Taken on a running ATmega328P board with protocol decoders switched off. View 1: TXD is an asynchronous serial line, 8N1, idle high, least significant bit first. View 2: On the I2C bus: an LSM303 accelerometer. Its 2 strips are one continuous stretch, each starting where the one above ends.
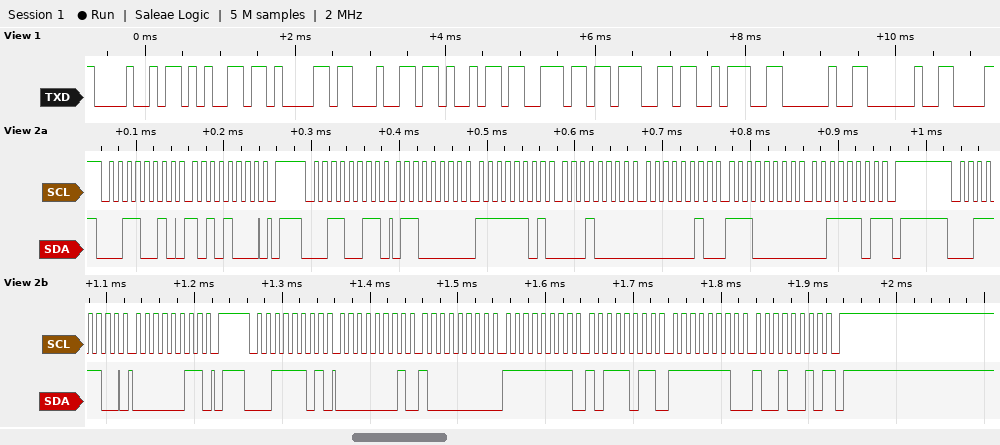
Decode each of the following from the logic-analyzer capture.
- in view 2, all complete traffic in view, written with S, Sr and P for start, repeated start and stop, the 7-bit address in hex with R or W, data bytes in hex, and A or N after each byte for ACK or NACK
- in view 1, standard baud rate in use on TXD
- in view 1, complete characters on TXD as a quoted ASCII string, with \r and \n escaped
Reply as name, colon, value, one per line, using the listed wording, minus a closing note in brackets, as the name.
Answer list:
in view 2, all complete traffic in view, written with S, Sr and P for start, repeated start and stop, the 7-bit address in hex with R or W, data bytes in hex, and A or N after each byte for ACK or NACK: S 19W A A8 A P S 19R A 60 A FD A 10 A 02 A E0 A 3D N P S 1EW A 03 A P S 1ER A 01 A 80 A FF A BB A FE A 92 N P
in view 1, standard baud rate in use on TXD: 9600 baud
in view 1, complete characters on TXD as a quoted ASCII string, with \r and \n escaped: "Heading:  "
